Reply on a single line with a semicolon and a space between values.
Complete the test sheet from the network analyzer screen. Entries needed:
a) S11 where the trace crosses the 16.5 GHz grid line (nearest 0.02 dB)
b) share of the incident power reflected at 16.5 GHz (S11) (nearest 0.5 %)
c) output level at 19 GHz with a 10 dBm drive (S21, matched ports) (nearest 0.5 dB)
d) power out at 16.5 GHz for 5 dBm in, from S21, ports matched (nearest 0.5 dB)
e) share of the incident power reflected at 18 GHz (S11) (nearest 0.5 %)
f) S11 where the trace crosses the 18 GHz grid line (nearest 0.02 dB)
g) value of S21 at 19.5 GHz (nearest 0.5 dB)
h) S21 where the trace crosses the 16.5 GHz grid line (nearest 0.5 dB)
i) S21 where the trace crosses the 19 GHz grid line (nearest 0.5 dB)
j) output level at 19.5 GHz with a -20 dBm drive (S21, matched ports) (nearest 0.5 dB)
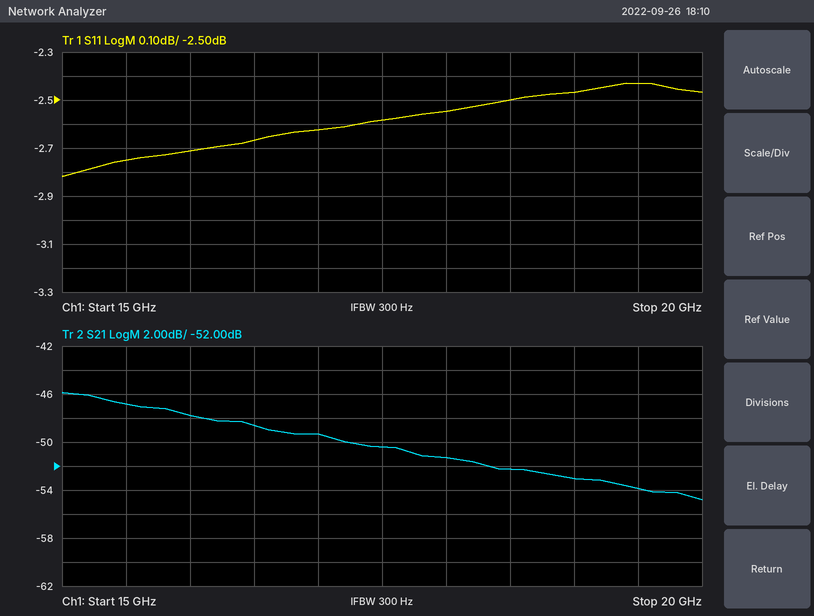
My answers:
-2.66 dB; 54.0 %; -43.0 dBm; -43.5 dBm; 55.5 %; -2.54 dB; -54.0 dB; -48.5 dB; -53.0 dB; -74.0 dBm
